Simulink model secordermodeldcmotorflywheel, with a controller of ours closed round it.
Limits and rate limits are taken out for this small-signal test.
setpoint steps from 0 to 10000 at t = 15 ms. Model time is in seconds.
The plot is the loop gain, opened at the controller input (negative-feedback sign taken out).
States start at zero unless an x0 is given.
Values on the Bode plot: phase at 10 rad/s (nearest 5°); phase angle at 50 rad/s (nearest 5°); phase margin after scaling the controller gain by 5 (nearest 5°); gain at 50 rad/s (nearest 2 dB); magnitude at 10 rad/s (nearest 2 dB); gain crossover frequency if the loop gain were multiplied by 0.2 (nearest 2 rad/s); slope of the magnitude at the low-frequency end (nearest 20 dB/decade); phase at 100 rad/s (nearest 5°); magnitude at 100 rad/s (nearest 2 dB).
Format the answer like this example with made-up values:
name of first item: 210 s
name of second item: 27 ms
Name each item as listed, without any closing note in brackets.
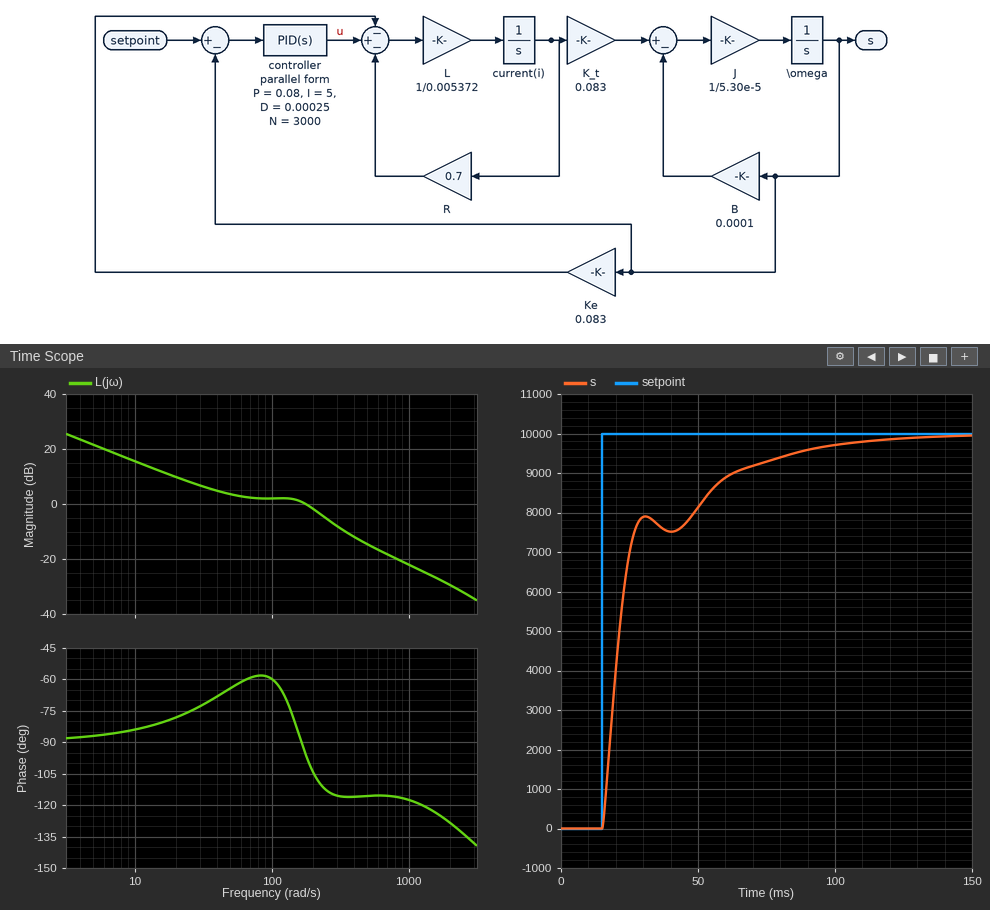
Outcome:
phase at 10 rad/s: -85°
phase angle at 50 rad/s: -65°
phase margin after scaling the controller gain by 5: 65°
gain at 50 rad/s: 4 dB
magnitude at 10 rad/s: 16 dB
gain crossover frequency if the loop gain were multiplied by 0.2: 12 rad/s
slope of the magnitude at the low-frequency end: -20 dB/decade
phase at 100 rad/s: -60°
magnitude at 100 rad/s: 2 dB
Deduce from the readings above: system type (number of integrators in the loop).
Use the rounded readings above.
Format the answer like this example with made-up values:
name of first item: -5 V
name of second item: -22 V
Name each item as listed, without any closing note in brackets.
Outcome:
system type: 1
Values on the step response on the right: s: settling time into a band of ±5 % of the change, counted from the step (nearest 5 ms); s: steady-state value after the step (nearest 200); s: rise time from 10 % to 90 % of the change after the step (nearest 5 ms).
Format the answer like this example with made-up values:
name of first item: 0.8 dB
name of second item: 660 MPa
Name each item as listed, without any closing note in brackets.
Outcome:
s: settling time into a band of ±5 % of the change, counted from the step: 70 ms
s: steady-state value after the step: 10000
s: rise time from 10 % to 90 % of the change after the step: 45 ms
